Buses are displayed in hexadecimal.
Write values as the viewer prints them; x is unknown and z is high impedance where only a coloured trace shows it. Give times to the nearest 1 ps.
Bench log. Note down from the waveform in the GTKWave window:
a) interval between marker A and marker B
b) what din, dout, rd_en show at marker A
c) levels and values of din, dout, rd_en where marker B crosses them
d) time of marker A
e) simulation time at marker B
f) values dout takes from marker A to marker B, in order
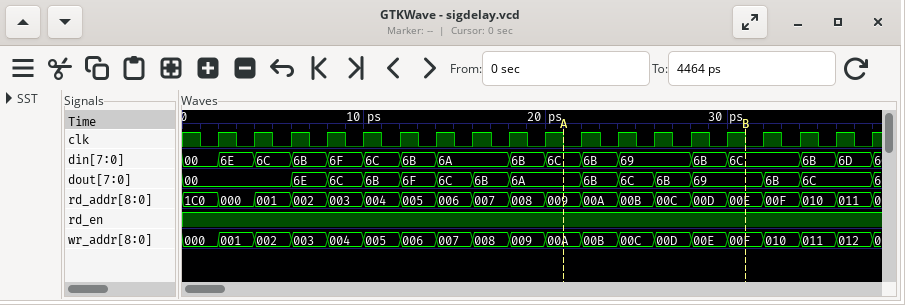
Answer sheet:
10 ps
din=6C, dout=6A, rd_en=1
din=6C, dout=69, rd_en=1
21 ps
31 ps
6A, 6B, 6C, 6B, 69
